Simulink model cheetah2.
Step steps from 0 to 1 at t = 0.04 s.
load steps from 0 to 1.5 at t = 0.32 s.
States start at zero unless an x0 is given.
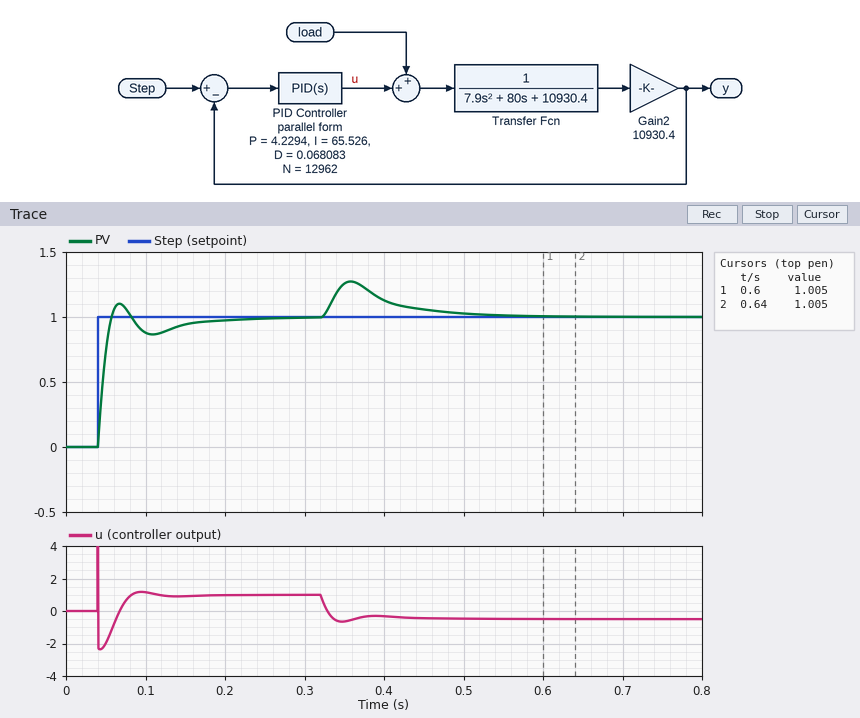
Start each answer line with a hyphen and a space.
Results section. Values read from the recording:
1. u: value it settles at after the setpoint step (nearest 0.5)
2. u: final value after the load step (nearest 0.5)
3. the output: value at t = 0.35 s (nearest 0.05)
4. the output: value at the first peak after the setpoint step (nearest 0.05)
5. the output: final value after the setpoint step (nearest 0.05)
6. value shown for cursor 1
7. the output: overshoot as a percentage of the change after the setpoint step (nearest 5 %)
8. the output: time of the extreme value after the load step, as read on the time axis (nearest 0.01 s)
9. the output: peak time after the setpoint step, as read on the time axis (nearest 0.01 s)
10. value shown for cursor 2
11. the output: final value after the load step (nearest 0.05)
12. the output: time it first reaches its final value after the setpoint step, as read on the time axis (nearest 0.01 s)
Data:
- 1.0
- -0.5
- 1.25
- 1.10
- 1.00
- 1.005
- 10 %
- 0.36 s
- 0.07 s
- 1.005
- 1.00
- 0.06 s
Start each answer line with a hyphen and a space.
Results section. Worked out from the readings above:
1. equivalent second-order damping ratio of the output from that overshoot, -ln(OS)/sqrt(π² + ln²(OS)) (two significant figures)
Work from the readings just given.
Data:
- 0.59
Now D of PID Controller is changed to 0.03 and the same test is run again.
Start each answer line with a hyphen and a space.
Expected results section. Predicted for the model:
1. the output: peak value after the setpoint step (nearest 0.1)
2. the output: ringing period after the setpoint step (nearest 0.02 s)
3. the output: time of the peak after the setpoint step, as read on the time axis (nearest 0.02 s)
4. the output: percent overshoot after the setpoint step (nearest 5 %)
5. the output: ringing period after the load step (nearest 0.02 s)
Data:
- 1.3
- 0.08 s
- 0.08 s
- 30 %
- 0.08 s
